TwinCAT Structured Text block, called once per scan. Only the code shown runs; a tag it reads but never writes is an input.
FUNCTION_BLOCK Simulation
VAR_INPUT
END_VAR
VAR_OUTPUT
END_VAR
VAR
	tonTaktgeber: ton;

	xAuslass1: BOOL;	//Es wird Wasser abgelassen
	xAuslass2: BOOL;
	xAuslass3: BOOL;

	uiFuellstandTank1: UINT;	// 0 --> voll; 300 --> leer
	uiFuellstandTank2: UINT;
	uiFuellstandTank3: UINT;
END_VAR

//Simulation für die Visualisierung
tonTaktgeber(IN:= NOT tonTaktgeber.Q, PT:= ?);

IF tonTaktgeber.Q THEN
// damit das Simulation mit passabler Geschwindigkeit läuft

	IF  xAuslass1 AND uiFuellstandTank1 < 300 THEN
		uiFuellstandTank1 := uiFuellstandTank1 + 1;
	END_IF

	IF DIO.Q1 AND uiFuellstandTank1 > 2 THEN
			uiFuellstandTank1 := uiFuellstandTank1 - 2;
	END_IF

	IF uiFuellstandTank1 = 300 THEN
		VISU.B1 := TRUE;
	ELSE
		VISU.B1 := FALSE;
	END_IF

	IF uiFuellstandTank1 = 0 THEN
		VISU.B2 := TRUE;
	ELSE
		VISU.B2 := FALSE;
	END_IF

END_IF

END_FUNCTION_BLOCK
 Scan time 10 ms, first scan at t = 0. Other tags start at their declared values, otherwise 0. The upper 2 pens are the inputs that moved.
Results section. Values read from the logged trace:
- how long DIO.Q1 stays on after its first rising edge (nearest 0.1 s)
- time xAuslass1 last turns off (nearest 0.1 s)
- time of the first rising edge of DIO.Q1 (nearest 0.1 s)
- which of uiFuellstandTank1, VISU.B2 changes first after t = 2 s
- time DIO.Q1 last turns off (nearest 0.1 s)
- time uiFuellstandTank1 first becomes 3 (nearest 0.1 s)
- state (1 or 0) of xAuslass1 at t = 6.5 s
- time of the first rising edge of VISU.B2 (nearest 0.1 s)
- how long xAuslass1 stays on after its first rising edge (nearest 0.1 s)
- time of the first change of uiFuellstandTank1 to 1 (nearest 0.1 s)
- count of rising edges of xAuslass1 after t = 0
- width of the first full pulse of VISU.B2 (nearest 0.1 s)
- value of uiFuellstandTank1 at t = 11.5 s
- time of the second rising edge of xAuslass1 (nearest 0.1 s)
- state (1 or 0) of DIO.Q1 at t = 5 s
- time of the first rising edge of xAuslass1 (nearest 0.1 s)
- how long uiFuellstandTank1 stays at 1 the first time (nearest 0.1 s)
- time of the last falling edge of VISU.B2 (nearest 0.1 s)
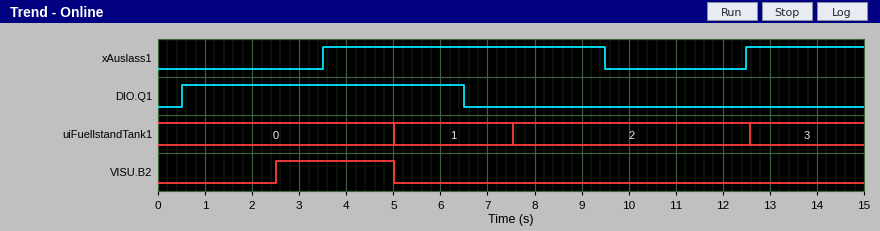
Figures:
6.0 s
9.5 s
0.5 s
VISU.B2
6.5 s
12.6 s
1
2.5 s
6.0 s
5.0 s
2
2.5 s
2
12.5 s
1
3.5 s
2.5 s
5.0 s
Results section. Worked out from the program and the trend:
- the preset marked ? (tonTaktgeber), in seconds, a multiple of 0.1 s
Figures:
2.5 s
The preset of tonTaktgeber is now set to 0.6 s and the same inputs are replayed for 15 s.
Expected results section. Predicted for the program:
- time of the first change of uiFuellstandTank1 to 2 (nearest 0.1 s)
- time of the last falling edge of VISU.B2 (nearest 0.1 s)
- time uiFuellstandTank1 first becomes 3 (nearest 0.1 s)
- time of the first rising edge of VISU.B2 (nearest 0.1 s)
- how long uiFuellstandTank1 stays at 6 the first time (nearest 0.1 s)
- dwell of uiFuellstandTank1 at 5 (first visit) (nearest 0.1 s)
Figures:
4.3 s
3.7 s
7.4 s
0.6 s
3.7 s
0.6 s
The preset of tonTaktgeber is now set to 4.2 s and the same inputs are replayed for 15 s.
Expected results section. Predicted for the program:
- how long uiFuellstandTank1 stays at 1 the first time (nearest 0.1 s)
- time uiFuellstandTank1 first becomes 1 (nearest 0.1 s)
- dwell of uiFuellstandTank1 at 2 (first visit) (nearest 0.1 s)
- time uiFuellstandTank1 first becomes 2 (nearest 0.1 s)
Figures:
4.2 s
4.2 s
4.2 s
8.4 s
